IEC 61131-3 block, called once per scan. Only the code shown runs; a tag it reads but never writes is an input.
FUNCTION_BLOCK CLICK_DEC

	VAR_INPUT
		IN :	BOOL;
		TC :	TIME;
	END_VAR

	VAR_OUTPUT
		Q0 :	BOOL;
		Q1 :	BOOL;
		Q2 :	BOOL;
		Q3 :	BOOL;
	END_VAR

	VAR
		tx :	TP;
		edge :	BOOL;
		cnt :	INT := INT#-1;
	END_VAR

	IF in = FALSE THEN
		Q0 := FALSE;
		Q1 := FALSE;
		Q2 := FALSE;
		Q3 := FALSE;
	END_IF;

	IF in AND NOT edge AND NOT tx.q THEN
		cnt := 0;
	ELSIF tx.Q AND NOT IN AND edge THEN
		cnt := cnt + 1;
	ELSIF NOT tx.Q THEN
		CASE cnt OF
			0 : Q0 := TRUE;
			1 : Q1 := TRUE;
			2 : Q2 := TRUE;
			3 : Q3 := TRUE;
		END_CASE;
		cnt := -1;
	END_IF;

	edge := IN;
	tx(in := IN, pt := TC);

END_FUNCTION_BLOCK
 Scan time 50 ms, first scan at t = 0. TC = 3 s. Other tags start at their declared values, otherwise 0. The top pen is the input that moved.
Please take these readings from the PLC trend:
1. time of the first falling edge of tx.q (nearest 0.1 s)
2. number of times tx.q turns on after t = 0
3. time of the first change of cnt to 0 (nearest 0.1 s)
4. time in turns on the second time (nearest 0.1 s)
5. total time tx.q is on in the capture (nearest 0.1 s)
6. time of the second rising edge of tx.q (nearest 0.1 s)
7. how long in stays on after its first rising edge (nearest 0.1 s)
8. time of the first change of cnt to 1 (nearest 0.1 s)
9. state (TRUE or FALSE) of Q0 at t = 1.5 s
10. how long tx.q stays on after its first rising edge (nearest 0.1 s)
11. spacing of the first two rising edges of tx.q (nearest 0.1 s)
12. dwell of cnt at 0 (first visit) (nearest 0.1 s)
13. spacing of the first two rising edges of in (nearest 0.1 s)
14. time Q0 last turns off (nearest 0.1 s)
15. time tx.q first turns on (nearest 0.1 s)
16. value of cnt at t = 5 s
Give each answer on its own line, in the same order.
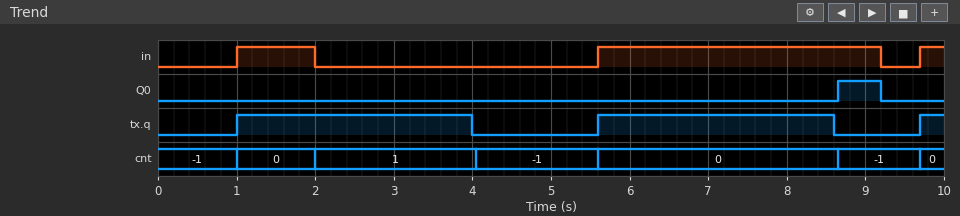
4.0 s
3
1.0 s
5.6 s
6.3 s
5.6 s
1.0 s
2.0 s
FALSE
3.0 s
4.6 s
1.0 s
4.6 s
9.2 s
1.0 s
-1
